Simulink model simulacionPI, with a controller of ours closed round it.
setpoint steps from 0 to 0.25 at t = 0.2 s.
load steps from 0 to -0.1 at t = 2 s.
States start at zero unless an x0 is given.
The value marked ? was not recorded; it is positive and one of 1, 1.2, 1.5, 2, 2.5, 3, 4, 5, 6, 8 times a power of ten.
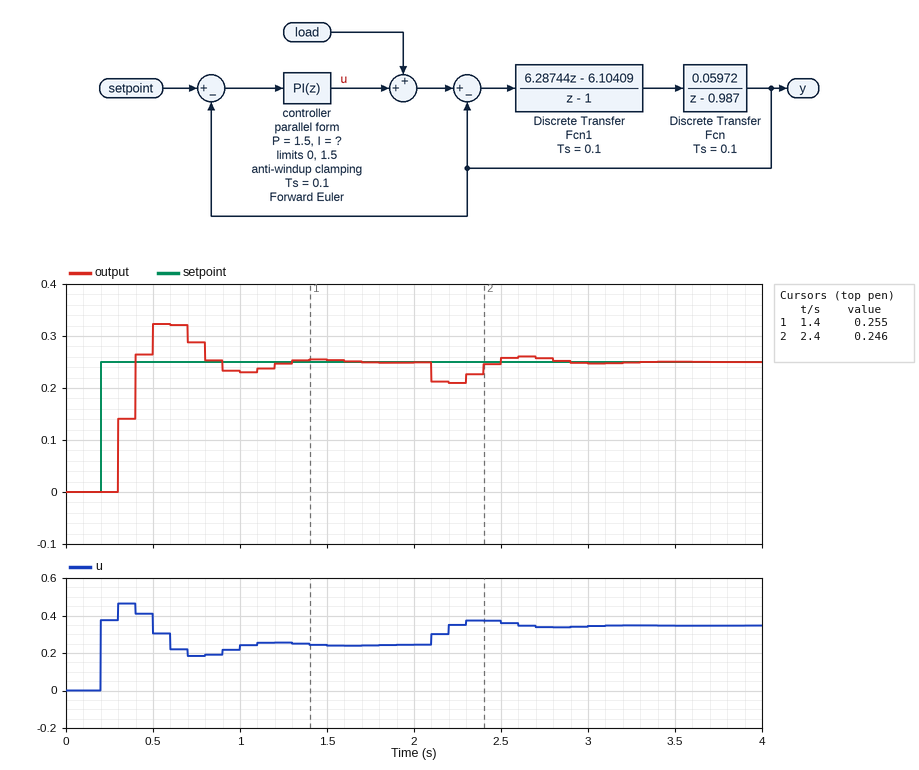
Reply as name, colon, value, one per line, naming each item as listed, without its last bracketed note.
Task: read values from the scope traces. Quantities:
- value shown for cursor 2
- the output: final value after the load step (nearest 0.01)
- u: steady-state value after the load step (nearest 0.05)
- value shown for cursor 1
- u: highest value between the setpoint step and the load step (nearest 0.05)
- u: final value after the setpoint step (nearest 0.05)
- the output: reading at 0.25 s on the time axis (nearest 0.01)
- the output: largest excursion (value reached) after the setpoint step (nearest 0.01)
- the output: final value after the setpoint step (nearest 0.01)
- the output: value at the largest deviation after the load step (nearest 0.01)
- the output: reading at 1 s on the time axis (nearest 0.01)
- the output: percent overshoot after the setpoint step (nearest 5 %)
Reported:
value shown for cursor 2: 0.246
the output: final value after the load step: 0.25
u: steady-state value after the load step: 0.35
value shown for cursor 1: 0.255
u: highest value between the setpoint step and the load step: 0.45
u: final value after the setpoint step: 0.25
the output: reading at 0.25 s on the time axis: 0.00
the output: largest excursion (value reached) after the setpoint step: 0.32
the output: final value after the setpoint step: 0.25
the output: value at the largest deviation after the load step: 0.21
the output: reading at 1 s on the time axis: 0.23
the output: percent overshoot after the setpoint step: 30 %
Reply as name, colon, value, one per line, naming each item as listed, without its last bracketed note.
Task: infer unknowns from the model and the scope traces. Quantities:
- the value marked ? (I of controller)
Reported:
the value marked ?: 12
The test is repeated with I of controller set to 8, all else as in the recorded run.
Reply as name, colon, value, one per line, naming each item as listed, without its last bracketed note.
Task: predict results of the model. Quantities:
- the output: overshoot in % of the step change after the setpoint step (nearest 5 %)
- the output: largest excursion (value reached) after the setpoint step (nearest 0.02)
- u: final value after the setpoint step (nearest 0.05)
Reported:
the output: overshoot in % of the step change after the setpoint step: 10 %
the output: largest excursion (value reached) after the setpoint step: 0.28
u: final value after the setpoint step: 0.25
